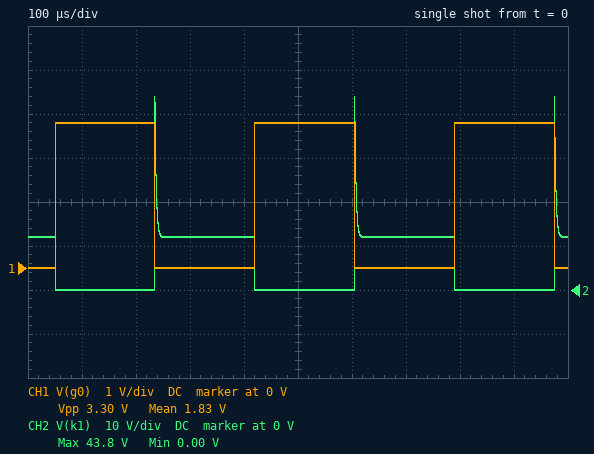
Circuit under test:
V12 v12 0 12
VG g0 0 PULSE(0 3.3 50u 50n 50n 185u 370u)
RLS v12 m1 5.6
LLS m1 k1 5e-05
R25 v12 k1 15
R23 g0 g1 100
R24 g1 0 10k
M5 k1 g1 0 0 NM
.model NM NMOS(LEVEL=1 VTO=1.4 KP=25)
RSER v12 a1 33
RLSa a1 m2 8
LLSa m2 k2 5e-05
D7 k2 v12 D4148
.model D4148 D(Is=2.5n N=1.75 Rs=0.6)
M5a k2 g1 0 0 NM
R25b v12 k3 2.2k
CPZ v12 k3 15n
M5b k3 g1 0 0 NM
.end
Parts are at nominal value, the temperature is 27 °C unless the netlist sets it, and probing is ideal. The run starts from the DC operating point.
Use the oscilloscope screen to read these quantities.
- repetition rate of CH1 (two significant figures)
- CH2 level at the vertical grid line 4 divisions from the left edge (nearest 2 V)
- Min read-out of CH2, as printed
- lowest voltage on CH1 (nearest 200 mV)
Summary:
2.7 kHz
12 V
0.00 V
0 V
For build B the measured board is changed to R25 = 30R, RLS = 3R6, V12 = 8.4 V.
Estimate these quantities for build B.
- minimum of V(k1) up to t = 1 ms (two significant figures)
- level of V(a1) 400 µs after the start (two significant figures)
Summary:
6.1 mV
8.4 V
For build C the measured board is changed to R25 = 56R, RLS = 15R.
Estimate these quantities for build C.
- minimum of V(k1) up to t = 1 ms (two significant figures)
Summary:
4.7 mV
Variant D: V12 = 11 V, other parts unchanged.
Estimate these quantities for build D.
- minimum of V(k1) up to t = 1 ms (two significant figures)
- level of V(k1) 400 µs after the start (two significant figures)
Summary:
16 mV
11 V
